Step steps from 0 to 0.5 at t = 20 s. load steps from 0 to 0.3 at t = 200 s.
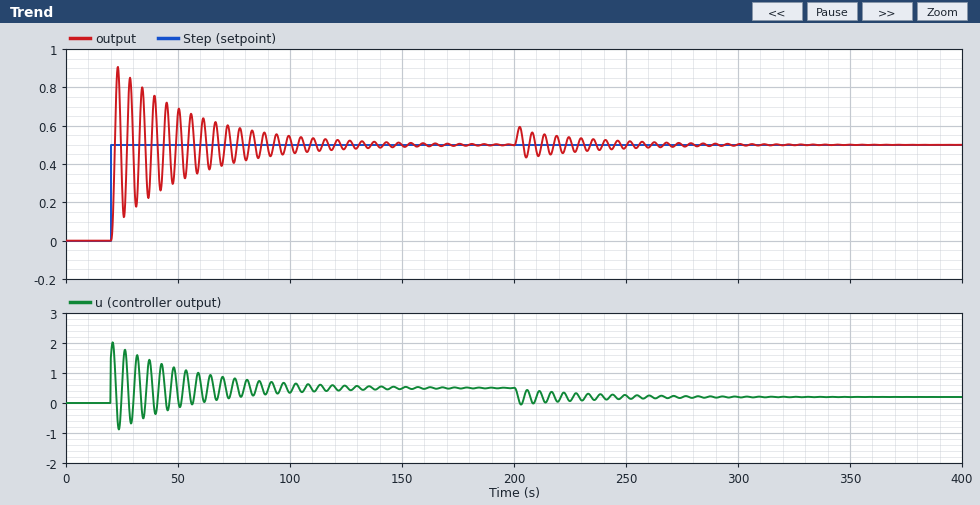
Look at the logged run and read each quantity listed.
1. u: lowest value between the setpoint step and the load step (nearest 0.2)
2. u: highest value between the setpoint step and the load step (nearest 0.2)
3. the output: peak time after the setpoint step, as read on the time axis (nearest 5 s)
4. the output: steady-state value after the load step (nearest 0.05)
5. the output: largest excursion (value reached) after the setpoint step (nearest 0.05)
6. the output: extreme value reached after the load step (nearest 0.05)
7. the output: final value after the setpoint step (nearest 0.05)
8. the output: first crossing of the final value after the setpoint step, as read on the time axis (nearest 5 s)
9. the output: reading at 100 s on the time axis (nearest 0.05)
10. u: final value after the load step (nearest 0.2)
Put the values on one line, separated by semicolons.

-0.8; 2.0; 25 s; 0.50; 0.90; 0.60; 0.50; 20 s; 0.55; 0.2
